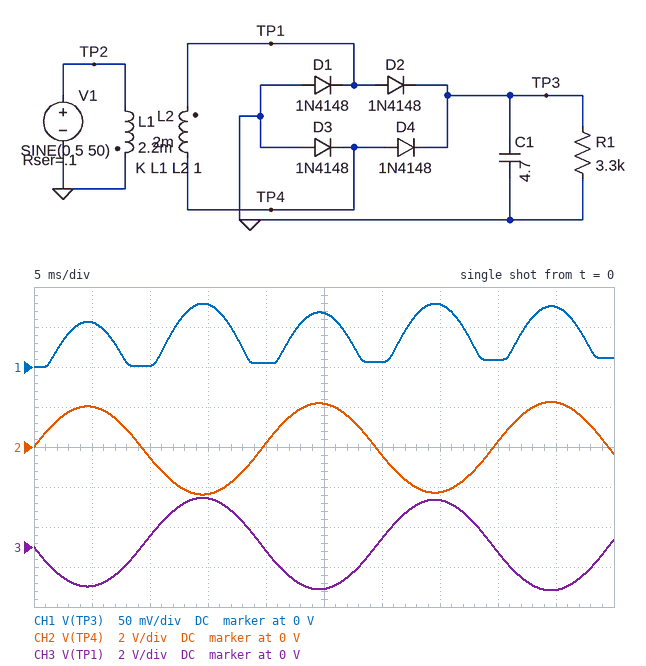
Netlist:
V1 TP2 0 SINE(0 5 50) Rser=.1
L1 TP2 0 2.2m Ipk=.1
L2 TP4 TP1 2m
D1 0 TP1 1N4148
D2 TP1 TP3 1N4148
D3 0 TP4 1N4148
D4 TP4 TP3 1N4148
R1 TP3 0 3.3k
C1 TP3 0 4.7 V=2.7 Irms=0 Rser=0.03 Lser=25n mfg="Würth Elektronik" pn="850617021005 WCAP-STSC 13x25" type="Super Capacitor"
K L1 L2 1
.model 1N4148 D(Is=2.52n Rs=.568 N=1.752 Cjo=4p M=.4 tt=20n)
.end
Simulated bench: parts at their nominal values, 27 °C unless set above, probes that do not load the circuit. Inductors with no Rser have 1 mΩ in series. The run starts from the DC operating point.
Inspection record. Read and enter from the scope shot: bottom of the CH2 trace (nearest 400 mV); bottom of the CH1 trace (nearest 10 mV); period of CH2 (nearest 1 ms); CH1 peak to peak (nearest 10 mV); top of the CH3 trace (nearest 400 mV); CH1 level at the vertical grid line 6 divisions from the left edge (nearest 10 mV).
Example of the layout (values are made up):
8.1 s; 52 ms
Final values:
-2.4 V; 0 V; 20 ms; 80 mV; 2.4 V; 10 mV
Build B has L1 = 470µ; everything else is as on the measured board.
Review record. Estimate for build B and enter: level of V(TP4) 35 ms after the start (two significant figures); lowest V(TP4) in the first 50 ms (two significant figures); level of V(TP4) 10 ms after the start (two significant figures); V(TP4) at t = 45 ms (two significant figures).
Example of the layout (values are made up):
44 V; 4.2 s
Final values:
-3.1 V; -3.7 V; -2.1 V; 3.2 V
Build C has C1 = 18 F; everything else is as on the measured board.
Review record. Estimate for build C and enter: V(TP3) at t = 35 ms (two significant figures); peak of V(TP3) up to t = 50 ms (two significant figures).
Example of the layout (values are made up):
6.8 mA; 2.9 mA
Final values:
72 mV; 77 mV
